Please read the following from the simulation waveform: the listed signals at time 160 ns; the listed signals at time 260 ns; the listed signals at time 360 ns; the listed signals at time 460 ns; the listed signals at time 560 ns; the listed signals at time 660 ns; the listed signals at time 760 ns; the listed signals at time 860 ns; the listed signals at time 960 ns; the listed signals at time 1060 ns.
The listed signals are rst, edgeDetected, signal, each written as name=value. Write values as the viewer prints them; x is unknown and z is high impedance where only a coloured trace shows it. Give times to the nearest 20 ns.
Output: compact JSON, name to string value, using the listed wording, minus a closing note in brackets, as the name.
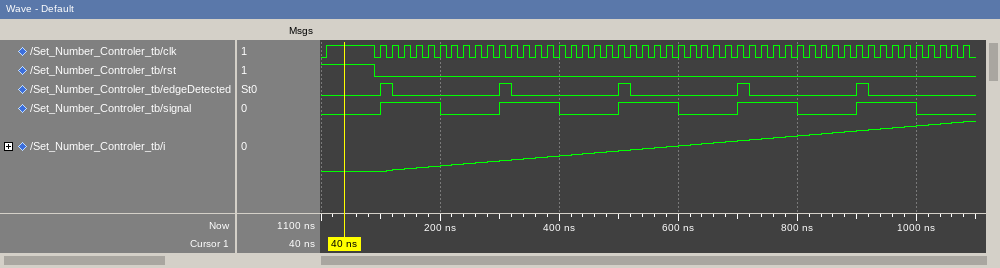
{"the listed signals at time 160 ns": "rst=0, edgeDetected=0, signal=1", "the listed signals at time 260 ns": "rst=0, edgeDetected=0, signal=0", "the listed signals at time 360 ns": "rst=0, edgeDetected=0, signal=1", "the listed signals at time 460 ns": "rst=0, edgeDetected=0, signal=0", "the listed signals at time 560 ns": "rst=0, edgeDetected=0, signal=1", "the listed signals at time 660 ns": "rst=0, edgeDetected=0, signal=0", "the listed signals at time 760 ns": "rst=0, edgeDetected=0, signal=1", "the listed signals at time 860 ns": "rst=0, edgeDetected=0, signal=0", "the listed signals at time 960 ns": "rst=0, edgeDetected=0, signal=1", "the listed signals at time 1060 ns": "rst=0, edgeDetected=0, signal=0"}
